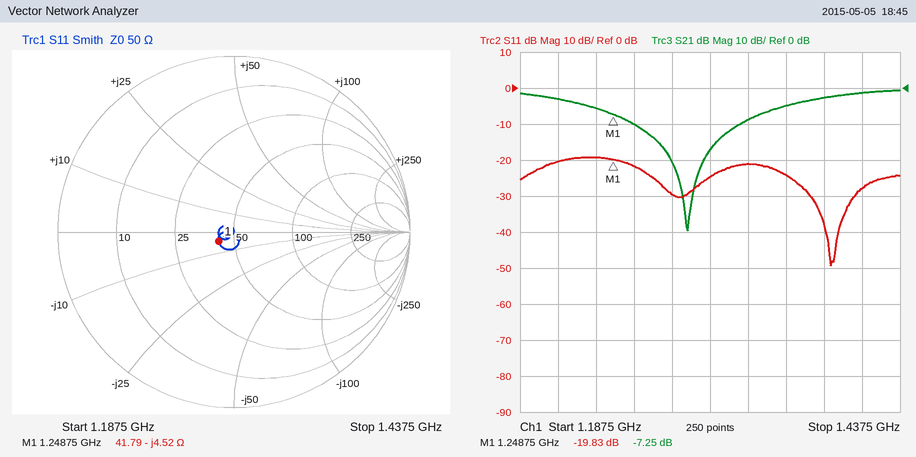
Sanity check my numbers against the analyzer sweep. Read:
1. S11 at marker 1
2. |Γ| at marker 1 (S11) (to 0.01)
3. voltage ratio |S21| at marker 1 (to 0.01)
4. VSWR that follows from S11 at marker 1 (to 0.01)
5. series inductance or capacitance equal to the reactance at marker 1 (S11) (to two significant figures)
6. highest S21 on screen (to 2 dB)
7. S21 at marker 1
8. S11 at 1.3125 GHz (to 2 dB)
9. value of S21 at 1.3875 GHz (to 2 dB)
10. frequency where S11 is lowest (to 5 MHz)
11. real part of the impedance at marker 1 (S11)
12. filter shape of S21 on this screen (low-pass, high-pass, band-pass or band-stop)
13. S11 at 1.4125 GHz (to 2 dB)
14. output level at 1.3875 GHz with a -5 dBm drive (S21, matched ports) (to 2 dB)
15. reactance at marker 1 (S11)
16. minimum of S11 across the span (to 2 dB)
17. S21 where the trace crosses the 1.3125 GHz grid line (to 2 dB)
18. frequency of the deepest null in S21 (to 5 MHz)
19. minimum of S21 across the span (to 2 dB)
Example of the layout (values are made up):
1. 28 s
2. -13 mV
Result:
1. -19.83 dB
2. 0.10
3. 0.43
4. 1.23
5. 28 pF
6. 0 dB
7. -7.25 dB
8. -24 dB
9. -2 dB
10. 1.390 GHz
11. 41.79 Ω
12. band-stop
13. -28 dB
14. -8 dBm
15. -4.52 Ω
16. -50 dB
17. -18 dB
18. 1.300 GHz
19. -40 dB
